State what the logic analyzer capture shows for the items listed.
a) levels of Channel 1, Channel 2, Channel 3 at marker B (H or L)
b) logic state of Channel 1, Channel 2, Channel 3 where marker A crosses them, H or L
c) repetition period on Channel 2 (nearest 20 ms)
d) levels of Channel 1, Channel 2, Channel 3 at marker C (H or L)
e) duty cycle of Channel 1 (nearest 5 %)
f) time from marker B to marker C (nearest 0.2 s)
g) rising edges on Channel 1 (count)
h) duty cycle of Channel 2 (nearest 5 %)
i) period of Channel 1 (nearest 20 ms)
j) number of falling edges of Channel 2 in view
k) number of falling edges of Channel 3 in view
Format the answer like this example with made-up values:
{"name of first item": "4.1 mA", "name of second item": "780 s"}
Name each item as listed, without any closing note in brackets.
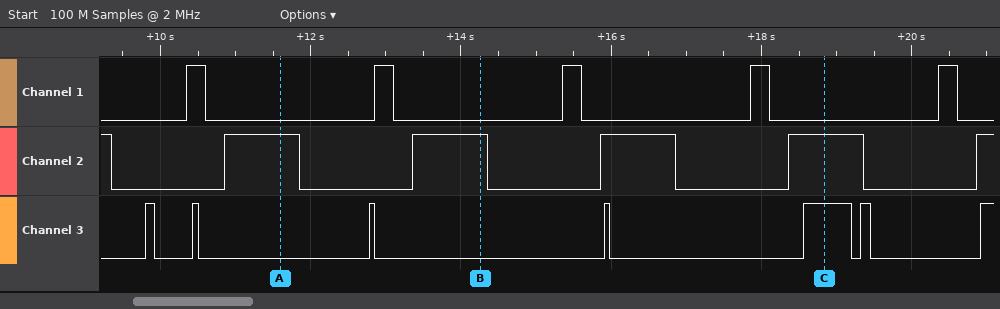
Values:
{"levels of Channel 1, Channel 2, Channel 3 at marker B": "Channel 1=L, Channel 2=H, Channel 3=L", "logic state of Channel 1, Channel 2, Channel 3 where marker A crosses them, H or L": "Channel 1=L, Channel 2=H, Channel 3=L", "repetition period on Channel 2": "2500 ms", "levels of Channel 1, Channel 2, Channel 3 at marker C": "Channel 1=L, Channel 2=H, Channel 3=H", "duty cycle of Channel 1": "10 %", "time from marker B to marker C": "4.6 s", "rising edges on Channel 1": "5", "duty cycle of Channel 2": "40 %", "period of Channel 1": "2500 ms", "number of falling edges of Channel 2 in view": "5", "number of falling edges of Channel 3 in view": "6"}
